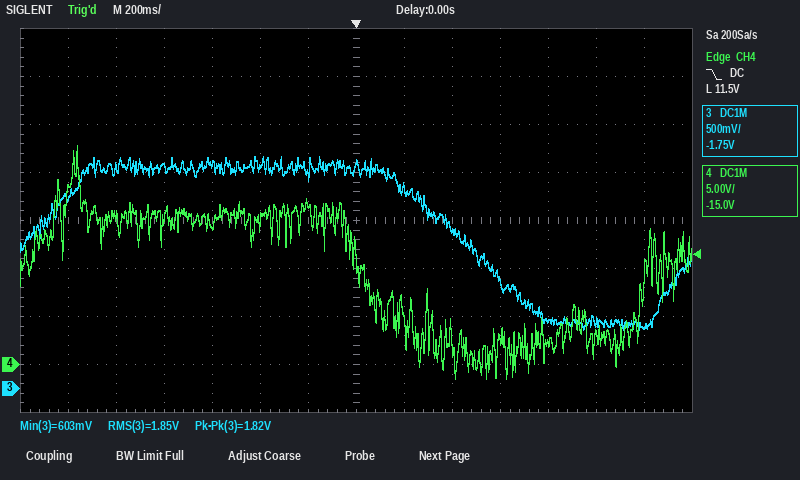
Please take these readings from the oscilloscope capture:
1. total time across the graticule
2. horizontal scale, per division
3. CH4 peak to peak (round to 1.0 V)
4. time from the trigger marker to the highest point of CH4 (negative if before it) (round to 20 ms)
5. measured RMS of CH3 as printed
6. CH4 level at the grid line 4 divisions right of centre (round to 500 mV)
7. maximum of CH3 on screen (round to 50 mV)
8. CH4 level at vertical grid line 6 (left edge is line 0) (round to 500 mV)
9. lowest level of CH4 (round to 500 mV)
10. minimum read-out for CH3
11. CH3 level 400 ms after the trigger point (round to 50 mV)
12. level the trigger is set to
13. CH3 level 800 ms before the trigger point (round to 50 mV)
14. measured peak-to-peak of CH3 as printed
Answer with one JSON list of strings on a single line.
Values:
["2.8 s", "200 ms", "24.0 V", "-1.16 s", "1.85 V", "2.5 V", "2.40 V", "17.0 V", "-1.5 V", "603 mV", "1.65 V", "11.5 V", "2.30 V", "1.82 V"]
